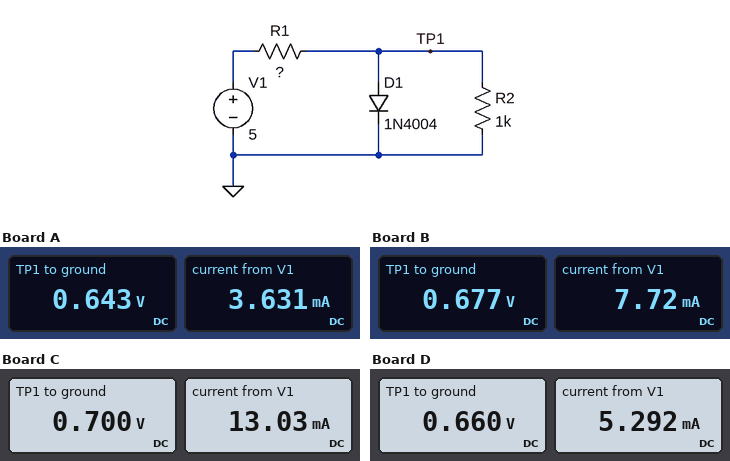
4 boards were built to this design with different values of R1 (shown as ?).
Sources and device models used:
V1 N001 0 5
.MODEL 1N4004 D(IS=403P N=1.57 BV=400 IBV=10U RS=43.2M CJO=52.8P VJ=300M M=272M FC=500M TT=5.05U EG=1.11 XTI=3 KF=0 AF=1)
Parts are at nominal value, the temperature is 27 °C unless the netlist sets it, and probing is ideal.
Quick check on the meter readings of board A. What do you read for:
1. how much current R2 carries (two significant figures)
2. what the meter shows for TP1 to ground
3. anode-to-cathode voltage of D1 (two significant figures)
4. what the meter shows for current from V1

640 µA
0.643 V
640 mV
3.631 mA
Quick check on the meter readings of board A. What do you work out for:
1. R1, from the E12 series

1.2 kΩ
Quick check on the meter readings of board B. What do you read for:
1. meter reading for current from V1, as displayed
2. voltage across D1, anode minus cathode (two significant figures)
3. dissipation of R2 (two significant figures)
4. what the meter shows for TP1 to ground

7.72 mA
680 mV
460 µW
0.677 V
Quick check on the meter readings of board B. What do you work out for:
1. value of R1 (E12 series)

560 Ω
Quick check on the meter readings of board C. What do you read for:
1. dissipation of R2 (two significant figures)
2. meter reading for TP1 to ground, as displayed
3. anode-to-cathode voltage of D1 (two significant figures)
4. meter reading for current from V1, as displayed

490 µW
0.700 V
700 mV
13.03 mA
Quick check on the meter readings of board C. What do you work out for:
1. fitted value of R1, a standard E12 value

330 Ω
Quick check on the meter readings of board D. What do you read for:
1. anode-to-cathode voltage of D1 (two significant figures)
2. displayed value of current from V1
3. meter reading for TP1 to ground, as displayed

660 mV
5.292 mA
0.660 V
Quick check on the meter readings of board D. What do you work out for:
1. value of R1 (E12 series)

820 Ω
